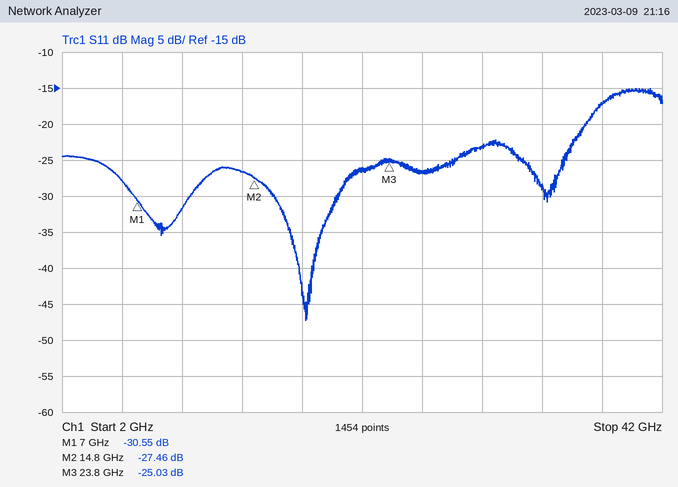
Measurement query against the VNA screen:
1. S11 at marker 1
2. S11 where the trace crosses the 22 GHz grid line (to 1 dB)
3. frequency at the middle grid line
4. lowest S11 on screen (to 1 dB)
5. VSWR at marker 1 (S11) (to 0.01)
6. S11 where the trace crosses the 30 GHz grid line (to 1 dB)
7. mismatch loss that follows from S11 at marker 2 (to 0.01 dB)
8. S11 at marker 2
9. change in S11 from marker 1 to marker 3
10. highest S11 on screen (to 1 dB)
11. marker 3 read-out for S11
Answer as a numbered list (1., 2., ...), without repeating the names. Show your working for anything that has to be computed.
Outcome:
1. -30.55 dB
2. -26 dB
3. 22 GHz
4. -47 dB
5. (1 + 0.0297)/(1 − 0.0297) ≈ 1.06
6. -23 dB
7. −10 log10(1 − 10^(-27.46/10)) ≈ 0.01 dB
8. -27.46 dB
9. -25.03 − (-30.55) = 5.52 dB
10. -15 dB
11. -25.03 dB
